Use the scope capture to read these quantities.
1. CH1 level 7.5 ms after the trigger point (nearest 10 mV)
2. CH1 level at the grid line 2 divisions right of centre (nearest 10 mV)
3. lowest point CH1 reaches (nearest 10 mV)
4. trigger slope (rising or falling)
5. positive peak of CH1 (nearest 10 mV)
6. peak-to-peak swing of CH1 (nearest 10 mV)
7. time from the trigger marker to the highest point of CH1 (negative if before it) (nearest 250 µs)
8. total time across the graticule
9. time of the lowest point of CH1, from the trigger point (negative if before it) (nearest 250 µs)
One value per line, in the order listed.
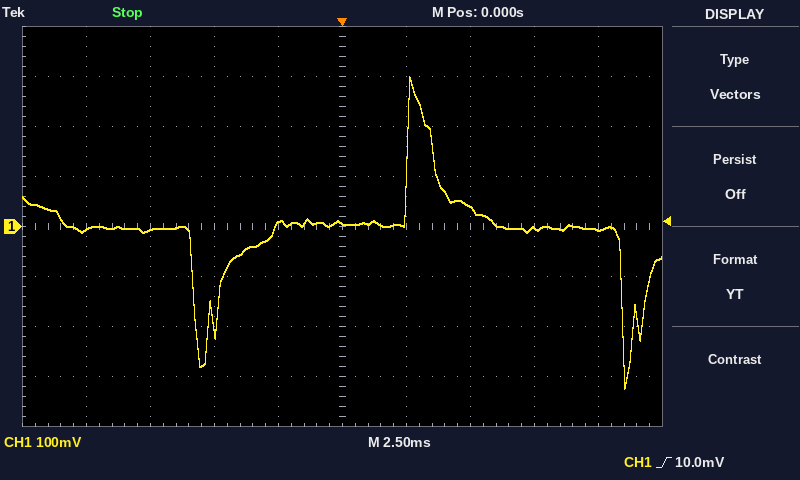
0 mV
40 mV
-320 mV
rising
300 mV
620 mV
+2.75 ms
25 ms
+11.00 ms
